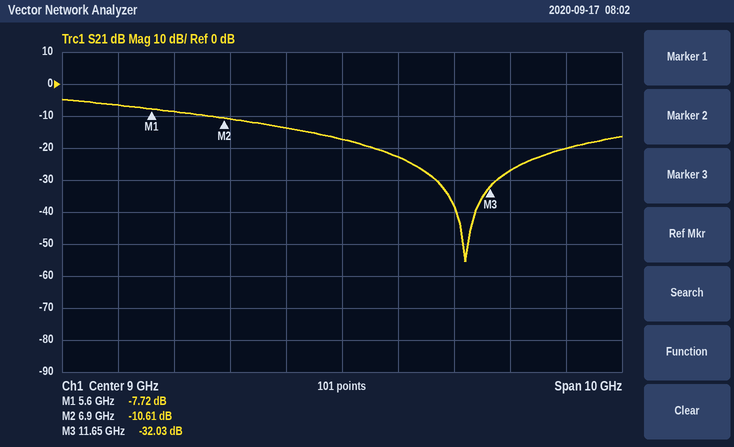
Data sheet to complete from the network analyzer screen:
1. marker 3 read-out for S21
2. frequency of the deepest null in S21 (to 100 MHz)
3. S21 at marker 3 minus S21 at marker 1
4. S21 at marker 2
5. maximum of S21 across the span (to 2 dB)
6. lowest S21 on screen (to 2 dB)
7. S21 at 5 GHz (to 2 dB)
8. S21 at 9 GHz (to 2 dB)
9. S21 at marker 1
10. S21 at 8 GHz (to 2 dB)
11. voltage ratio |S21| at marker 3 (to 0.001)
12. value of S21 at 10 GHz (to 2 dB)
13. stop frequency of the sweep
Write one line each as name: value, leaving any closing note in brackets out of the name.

marker 3 read-out for S21: -32.03 dB
frequency of the deepest null in S21: 11.2 GHz
S21 at marker 3 minus S21 at marker 1: -24.31 dB
S21 at marker 2: -10.61 dB
maximum of S21 across the span: -4 dB
lowest S21 on screen: -56 dB
S21 at 5 GHz: -6 dB
S21 at 9 GHz: -18 dB
S21 at marker 1: -7.72 dB
S21 at 8 GHz: -14 dB
voltage ratio |S21| at marker 3: 0.025
value of S21 at 10 GHz: -22 dB
stop frequency of the sweep: 14 GHz
